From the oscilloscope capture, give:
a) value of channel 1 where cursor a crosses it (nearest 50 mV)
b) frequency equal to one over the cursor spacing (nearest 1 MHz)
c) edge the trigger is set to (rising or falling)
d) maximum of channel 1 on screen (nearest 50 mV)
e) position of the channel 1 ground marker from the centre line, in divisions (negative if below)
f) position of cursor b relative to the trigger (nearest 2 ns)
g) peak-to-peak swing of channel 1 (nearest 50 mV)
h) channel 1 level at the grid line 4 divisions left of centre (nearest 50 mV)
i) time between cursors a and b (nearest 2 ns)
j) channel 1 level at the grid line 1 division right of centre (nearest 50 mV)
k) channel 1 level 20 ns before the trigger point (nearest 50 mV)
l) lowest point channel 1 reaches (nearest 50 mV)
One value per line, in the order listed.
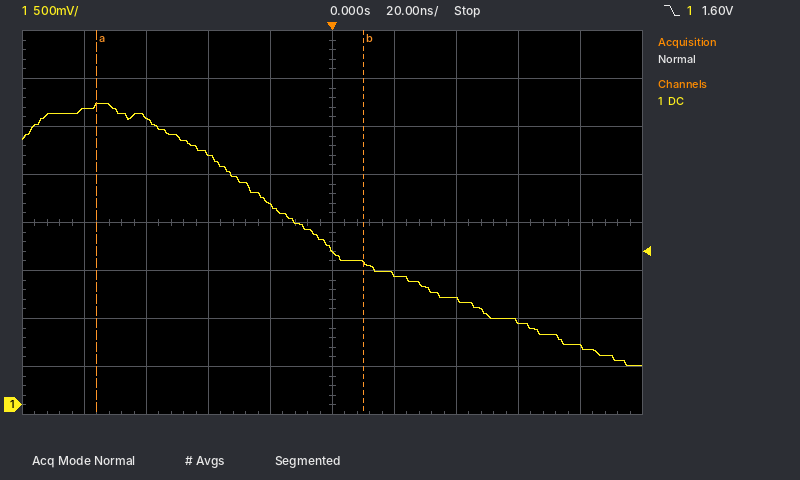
3.10 V
12 MHz
falling
3.15 V
-3.8 div
+10 ns
2.75 V
3.10 V
86 ns
1.35 V
2.10 V
400 mV
